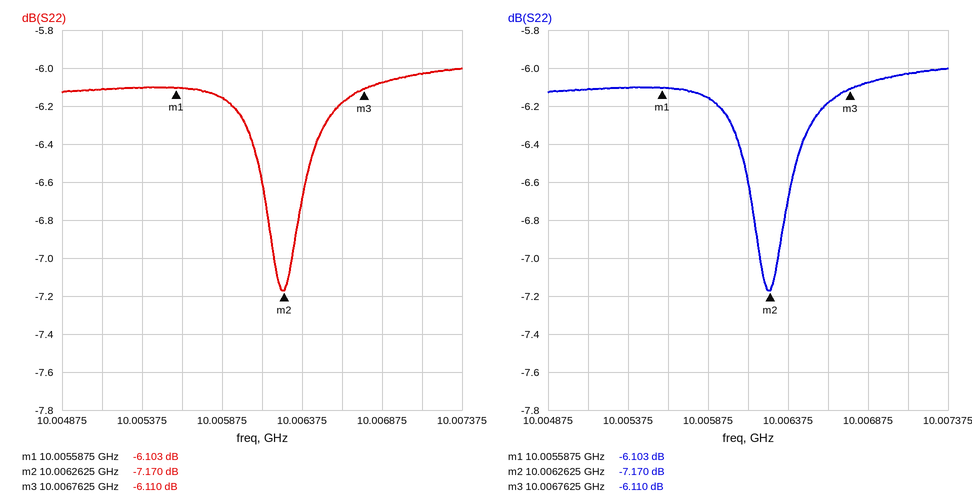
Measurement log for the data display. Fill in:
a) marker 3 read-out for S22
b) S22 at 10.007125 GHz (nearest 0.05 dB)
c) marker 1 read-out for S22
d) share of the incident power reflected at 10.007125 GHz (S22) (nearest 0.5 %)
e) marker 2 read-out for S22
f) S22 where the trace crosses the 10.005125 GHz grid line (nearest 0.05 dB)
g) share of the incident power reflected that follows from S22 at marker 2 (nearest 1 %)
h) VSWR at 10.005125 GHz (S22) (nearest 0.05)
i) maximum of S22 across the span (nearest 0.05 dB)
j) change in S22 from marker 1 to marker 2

-6.110 dB
-6.05 dB
-6.103 dB
25.0 %
-7.170 dB
-6.10 dB
19 %
2.95
-6.00 dB
-1.067 dB
